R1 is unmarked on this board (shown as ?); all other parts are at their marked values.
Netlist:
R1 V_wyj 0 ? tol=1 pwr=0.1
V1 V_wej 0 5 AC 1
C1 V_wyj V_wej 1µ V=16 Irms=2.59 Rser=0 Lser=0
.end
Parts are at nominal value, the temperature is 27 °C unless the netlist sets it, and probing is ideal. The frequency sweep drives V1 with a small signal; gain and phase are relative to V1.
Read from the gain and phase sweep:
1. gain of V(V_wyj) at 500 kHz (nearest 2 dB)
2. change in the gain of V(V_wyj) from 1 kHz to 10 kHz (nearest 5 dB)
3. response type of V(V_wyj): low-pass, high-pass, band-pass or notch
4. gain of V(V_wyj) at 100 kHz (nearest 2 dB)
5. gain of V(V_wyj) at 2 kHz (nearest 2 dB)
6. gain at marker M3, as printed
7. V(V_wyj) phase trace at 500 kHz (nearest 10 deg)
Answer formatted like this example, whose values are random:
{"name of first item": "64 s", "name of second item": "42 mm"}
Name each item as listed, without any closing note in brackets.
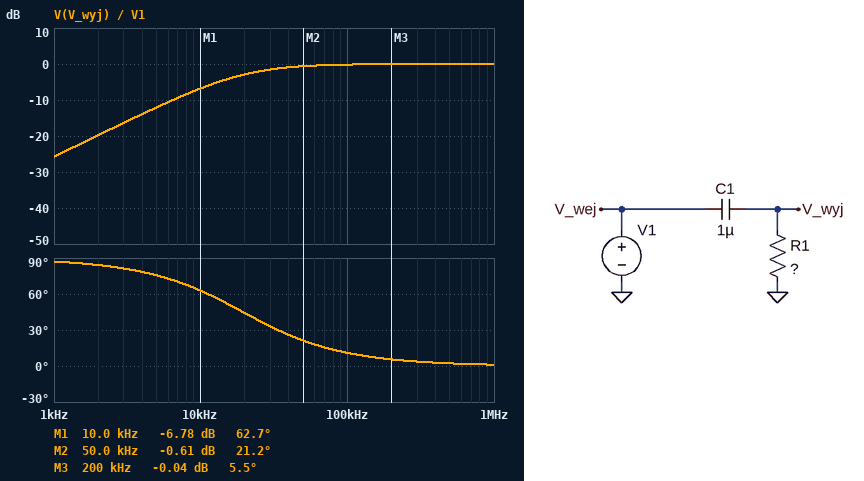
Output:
{"gain of V(V_wyj) at 500 kHz": "0 dB", "change in the gain of V(V_wyj) from 1 kHz to 10 kHz": "20 dB", "response type of V(V_wyj): low-pass, high-pass, band-pass or notch": "high-pass", "gain of V(V_wyj) at 100 kHz": "0 dB", "gain of V(V_wyj) at 2 kHz": "-20 dB", "gain at marker M3, as printed": "-0.04 dB", "V(V_wyj) phase trace at 500 kHz": "0 deg"}
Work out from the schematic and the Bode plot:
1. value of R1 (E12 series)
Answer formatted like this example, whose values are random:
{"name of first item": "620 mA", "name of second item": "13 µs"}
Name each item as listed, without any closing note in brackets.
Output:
{"value of R1": "8.2 Ω"}
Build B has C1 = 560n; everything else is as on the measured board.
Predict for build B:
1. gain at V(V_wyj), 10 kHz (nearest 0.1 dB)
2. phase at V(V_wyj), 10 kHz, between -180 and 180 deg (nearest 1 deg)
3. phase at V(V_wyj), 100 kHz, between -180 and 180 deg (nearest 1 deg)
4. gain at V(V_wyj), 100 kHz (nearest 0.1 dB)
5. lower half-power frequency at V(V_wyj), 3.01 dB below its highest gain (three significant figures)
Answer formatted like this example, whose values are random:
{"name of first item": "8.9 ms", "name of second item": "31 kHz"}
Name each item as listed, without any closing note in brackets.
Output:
{"gain at V(V_wyj), 10 kHz": "-11.1 dB", "phase at V(V_wyj), 10 kHz, between -180 and 180 deg": "74 deg", "phase at V(V_wyj), 100 kHz, between -180 and 180 deg": "19 deg", "gain at V(V_wyj), 100 kHz": "-0.5 dB", "lower half-power frequency at V(V_wyj), 3.01 dB below its highest gain": "34.7 kHz"}
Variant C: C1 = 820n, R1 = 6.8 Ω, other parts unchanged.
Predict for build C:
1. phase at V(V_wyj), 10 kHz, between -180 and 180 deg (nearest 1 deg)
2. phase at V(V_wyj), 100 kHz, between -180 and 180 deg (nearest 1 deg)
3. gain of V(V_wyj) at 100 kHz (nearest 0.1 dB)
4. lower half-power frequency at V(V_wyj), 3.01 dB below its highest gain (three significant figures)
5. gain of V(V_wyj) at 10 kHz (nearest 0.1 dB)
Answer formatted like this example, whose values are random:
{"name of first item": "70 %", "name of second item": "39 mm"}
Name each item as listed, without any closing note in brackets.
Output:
{"phase at V(V_wyj), 10 kHz, between -180 and 180 deg": "71 deg", "phase at V(V_wyj), 100 kHz, between -180 and 180 deg": "16 deg", "gain of V(V_wyj) at 100 kHz": "-0.3 dB", "lower half-power frequency at V(V_wyj), 3.01 dB below its highest gain": "28.5 kHz", "gain of V(V_wyj) at 10 kHz": "-9.6 dB"}
